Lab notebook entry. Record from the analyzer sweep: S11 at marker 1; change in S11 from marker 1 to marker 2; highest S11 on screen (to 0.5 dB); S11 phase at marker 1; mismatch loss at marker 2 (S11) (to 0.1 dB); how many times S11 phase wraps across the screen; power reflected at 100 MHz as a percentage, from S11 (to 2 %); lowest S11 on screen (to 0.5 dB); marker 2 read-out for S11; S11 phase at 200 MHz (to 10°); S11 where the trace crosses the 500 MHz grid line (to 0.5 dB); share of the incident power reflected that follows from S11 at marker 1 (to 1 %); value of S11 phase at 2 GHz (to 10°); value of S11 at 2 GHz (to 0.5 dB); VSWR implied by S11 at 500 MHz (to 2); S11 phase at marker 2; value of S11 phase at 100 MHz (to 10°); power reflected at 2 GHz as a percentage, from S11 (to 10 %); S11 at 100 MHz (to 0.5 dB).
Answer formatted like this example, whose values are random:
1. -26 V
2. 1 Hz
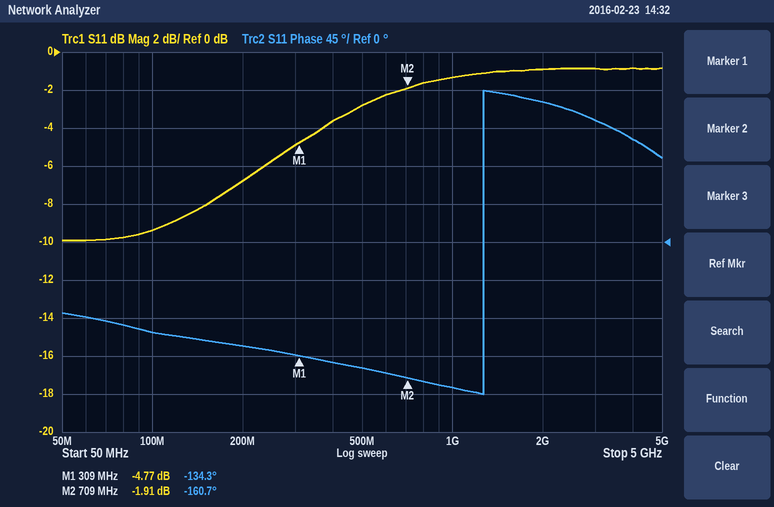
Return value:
1. -4.77 dB
2. 2.86 dB
3. -1.0 dB
4. -134.3°
5. 4.5 dB
6. 1
7. 12 %
8. -10.0 dB
9. -1.91 dB
10. -120°
11. -3.0 dB
12. 33 %
13. 170°
14. -1.0 dB
15. 6
16. -160.7°
17. -110°
18. 80 %
19. -9.5 dB
